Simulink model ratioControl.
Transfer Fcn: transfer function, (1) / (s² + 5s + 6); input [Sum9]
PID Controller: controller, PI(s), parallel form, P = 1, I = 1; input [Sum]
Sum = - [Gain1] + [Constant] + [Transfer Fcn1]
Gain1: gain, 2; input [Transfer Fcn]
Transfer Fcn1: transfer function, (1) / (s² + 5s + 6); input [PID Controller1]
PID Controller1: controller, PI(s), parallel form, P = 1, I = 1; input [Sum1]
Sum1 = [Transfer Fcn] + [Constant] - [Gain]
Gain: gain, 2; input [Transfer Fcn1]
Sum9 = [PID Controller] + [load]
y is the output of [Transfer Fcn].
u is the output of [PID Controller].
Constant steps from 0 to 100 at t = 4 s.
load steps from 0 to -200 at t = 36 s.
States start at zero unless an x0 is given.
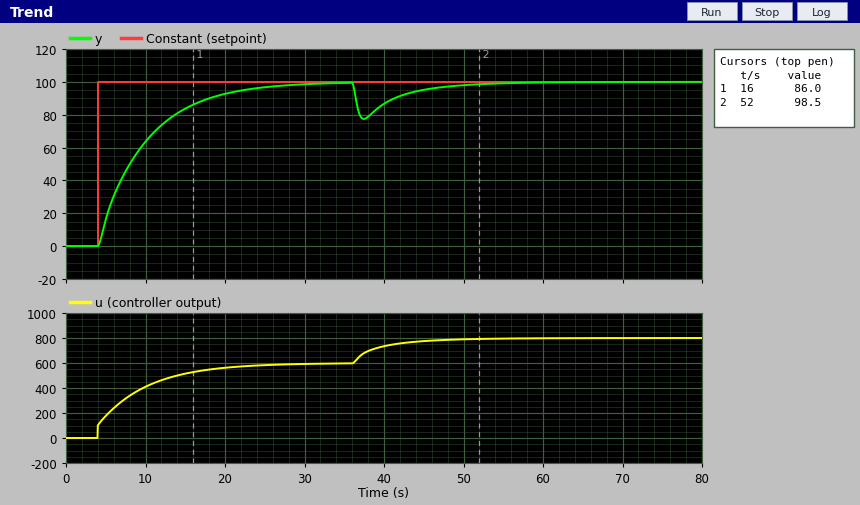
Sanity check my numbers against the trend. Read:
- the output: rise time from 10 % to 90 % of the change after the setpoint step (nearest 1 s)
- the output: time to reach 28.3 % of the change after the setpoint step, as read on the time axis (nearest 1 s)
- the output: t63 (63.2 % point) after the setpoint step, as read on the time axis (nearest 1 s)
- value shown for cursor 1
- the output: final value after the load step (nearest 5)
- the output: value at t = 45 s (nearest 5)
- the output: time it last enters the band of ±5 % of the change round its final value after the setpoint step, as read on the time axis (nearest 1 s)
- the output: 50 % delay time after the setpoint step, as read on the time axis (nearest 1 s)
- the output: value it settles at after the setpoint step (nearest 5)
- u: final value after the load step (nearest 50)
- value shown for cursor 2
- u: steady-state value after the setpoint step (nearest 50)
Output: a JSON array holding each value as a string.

["13 s", "6 s", "10 s", "86.0", "100", "95", "22 s", "8 s", "100", "800", "98.5", "600"]
